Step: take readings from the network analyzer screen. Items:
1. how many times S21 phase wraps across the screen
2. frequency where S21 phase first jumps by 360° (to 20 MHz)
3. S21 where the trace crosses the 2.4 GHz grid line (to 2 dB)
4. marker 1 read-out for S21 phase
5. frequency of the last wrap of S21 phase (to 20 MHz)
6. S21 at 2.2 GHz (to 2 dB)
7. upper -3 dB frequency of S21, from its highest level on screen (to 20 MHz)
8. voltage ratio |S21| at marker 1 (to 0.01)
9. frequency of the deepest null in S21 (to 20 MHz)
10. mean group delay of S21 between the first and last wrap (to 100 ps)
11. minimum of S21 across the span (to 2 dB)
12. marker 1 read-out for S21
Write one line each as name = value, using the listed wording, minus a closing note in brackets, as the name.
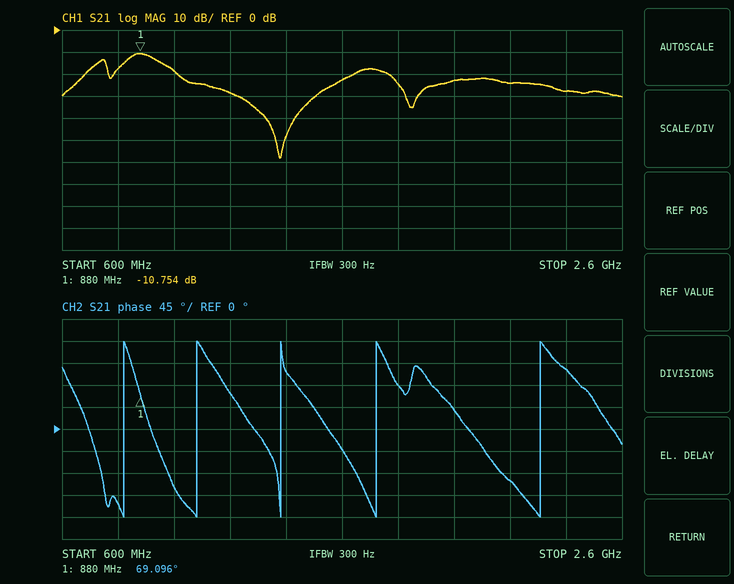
how many times S21 phase wraps across the screen = 5
frequency where S21 phase first jumps by 360° = 820 MHz
S21 where the trace crosses the 2.4 GHz grid line = -28 dB
marker 1 read-out for S21 phase = 69.096°
frequency of the last wrap of S21 phase = 2.30 GHz
S21 at 2.2 GHz = -24 dB
upper -3 dB frequency of S21, from its highest level on screen = 940 MHz
voltage ratio |S21| at marker 1 = 0.29
frequency of the deepest null in S21 = 1.38 GHz
mean group delay of S21 between the first and last wrap = 2.7 ns
minimum of S21 across the span = -58 dB
marker 1 read-out for S21 = -10.754 dB
